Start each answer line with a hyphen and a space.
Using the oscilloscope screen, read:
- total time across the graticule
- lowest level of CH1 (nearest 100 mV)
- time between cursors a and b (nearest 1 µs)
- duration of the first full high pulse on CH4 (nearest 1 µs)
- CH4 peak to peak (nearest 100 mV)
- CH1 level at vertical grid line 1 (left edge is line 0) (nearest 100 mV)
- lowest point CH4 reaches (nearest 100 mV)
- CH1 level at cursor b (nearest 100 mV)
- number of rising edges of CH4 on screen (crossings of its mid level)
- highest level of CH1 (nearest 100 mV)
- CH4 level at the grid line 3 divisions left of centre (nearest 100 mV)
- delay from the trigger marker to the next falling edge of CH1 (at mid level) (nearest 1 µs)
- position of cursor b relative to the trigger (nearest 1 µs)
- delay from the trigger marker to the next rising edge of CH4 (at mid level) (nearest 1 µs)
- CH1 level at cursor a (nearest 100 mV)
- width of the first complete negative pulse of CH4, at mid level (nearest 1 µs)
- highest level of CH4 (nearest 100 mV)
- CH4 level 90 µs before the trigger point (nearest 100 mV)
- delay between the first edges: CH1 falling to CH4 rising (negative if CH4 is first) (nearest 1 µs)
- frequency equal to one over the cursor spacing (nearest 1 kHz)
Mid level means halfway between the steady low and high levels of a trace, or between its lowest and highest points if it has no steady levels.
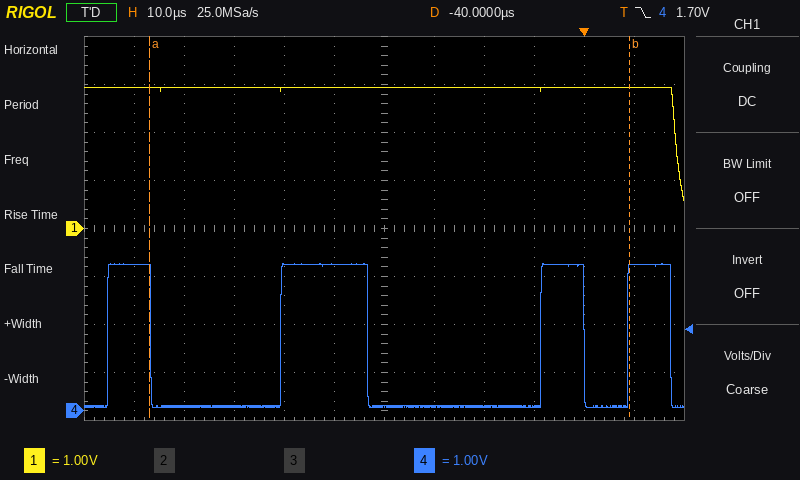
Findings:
- 120 µs
- 600 mV
- 96 µs
- 9 µs
- 3.0 V
- 2.9 V
- 100 mV
- 2.9 V
- 4
- 2.9 V
- 100 mV
- 18 µs
- +9 µs
- 9 µs
- 2.9 V
- 26 µs
- 3.1 V
- 3.0 V
- -114 µs
- 10 kHz
